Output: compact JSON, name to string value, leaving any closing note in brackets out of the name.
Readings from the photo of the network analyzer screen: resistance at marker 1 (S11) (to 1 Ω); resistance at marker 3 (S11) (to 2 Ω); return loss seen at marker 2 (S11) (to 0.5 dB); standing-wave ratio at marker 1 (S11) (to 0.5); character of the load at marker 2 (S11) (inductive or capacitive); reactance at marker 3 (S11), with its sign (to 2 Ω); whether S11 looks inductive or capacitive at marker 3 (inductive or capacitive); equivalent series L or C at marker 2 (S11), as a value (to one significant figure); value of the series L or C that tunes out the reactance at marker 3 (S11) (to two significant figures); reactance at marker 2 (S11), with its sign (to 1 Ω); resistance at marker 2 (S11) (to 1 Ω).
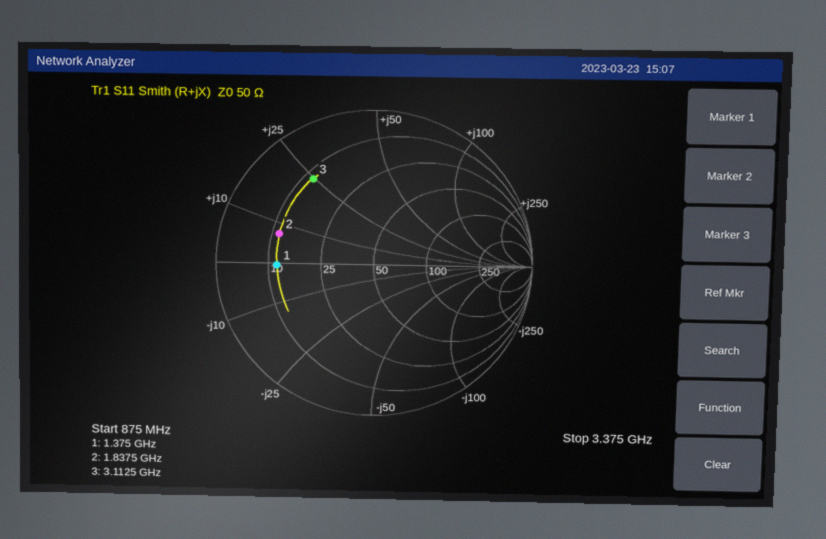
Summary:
{"resistance at marker 1 (S11)": "12 Ω", "resistance at marker 3 (S11)": "12 Ω", "return loss seen at marker 2 (S11)": "4.0 dB", "standing-wave ratio at marker 1 (S11)": "4.0", "character of the load at marker 2 (S11)": "inductive", "reactance at marker 3 (S11), with its sign": "+24 Ω", "whether S11 looks inductive or capacitive at marker 3": "inductive", "equivalent series L or C at marker 2 (S11), as a value": "600 pH", "value of the series L or C that tunes out the reactance at marker 3 (S11)": "2.1 pF", "reactance at marker 2 (S11), with its sign": "+7 Ω", "resistance at marker 2 (S11)": "12 Ω"}
